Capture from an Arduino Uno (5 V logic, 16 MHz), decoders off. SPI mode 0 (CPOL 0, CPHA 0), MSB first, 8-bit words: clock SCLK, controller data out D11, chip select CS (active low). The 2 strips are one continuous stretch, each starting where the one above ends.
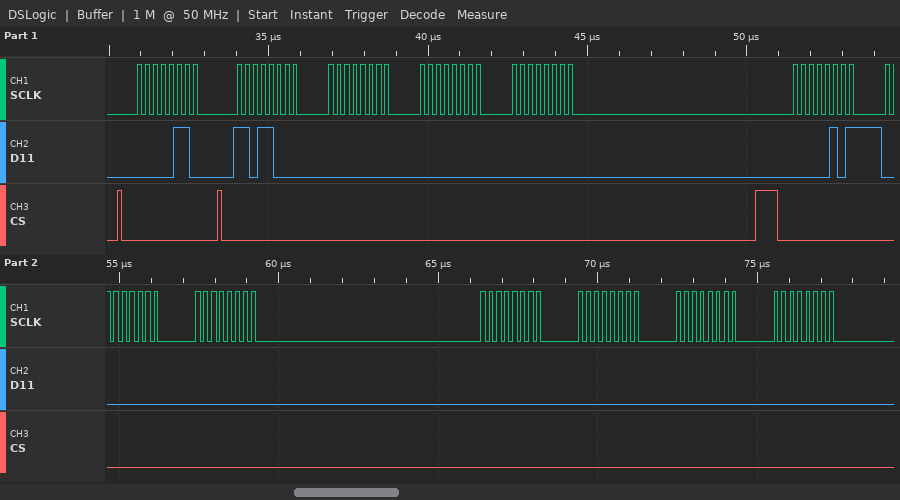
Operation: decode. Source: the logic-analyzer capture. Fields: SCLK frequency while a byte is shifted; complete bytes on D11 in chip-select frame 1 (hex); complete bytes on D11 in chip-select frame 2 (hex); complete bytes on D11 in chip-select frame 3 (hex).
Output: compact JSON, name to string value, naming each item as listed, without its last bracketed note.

{"SCLK frequency while a byte is shifted": "4 MHz", "complete bytes on D11 in chip-select frame 1": "06", "complete bytes on D11 in chip-select frame 2": "D8 00 00 00", "complete bytes on D11 in chip-select frame 3": "05 00 00 00 00 00 00"}
